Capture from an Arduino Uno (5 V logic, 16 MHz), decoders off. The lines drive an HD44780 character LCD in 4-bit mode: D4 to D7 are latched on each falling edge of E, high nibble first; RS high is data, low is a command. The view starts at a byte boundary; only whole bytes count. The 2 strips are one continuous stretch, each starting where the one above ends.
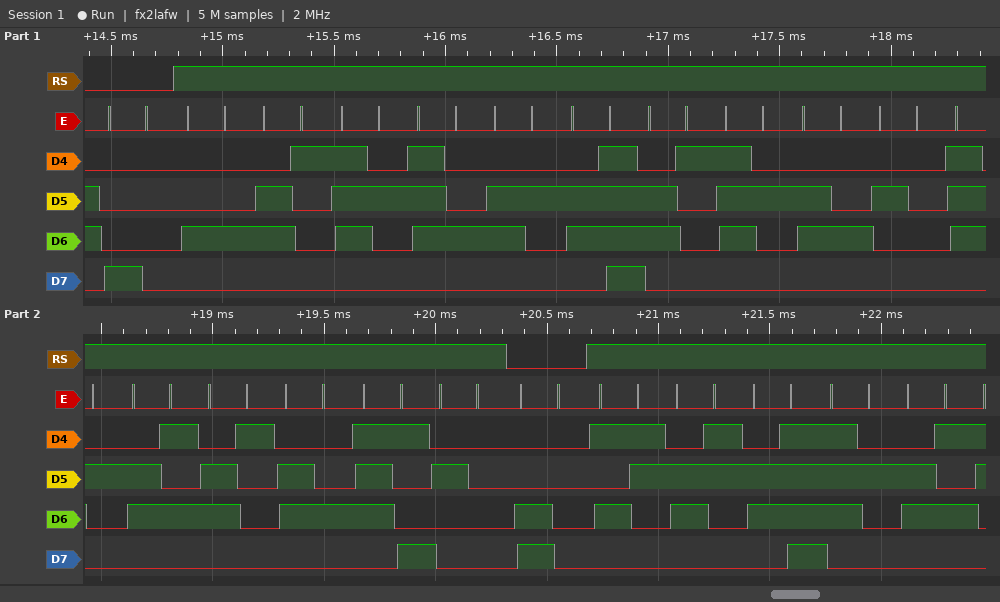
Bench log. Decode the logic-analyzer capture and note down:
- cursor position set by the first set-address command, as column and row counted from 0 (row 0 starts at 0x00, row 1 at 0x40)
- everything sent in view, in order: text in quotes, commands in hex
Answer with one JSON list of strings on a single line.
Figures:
["column 0, row 0", "0x80 \"Dartboard ready \" 0xC0 \"Score\""]
